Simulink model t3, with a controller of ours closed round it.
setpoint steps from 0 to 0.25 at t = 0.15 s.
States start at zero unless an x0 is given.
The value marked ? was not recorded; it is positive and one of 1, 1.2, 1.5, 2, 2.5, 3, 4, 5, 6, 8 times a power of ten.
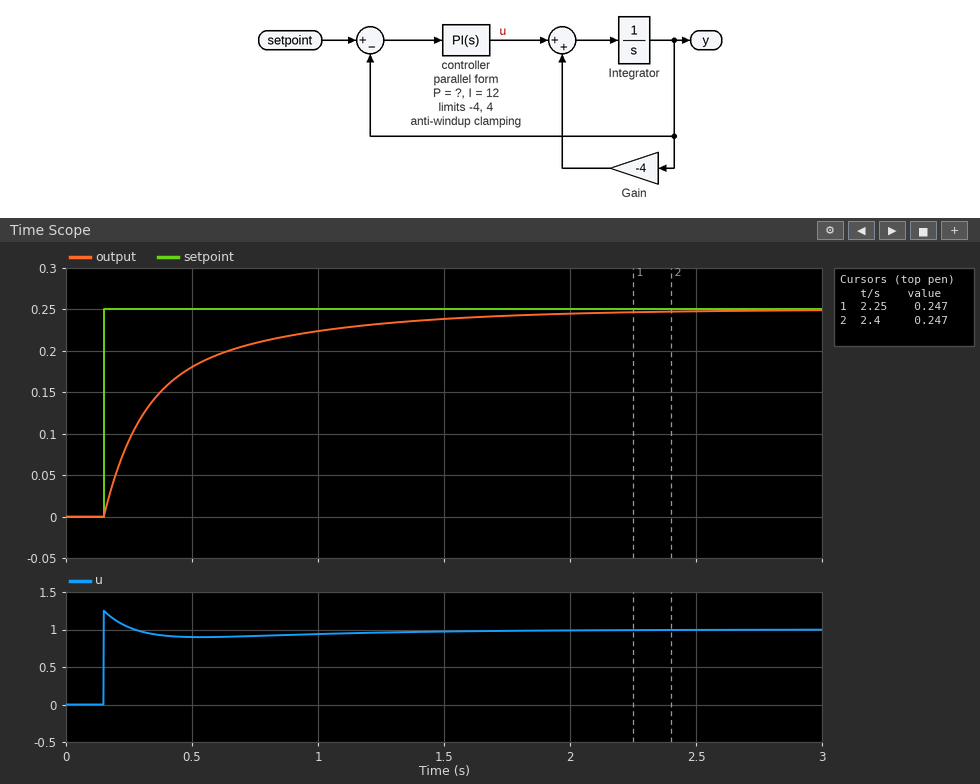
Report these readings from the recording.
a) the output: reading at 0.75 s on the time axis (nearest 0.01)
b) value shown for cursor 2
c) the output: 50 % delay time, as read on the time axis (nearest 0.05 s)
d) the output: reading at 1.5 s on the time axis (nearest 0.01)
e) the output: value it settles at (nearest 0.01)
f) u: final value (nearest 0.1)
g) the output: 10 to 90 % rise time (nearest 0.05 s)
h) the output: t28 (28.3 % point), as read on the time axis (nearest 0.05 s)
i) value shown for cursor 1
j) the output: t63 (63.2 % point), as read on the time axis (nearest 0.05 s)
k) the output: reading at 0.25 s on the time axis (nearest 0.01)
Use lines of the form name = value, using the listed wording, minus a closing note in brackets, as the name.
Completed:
the output: reading at 0.75 s on the time axis = 0.21
value shown for cursor 2 = 0.247
the output: 50 % delay time, as read on the time axis = 0.30 s
the output: reading at 1.5 s on the time axis = 0.24
the output: value it settles at = 0.25
u: final value = 1.0
the output: 10 to 90 % rise time = 0.85 s
the output: t28 (28.3 % point), as read on the time axis = 0.20 s
value shown for cursor 1 = 0.247
the output: t63 (63.2 % point), as read on the time axis = 0.40 s
the output: reading at 0.25 s on the time axis = 0.09
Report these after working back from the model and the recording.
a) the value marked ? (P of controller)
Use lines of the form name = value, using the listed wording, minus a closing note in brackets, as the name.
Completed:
the value marked ? = 5
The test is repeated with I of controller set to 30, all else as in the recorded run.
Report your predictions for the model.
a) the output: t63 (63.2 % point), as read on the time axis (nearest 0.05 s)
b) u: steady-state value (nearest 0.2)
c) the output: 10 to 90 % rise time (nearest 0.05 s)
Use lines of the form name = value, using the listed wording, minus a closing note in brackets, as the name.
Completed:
the output: t63 (63.2 % point), as read on the time axis = 0.30 s
u: steady-state value = 1.0
the output: 10 to 90 % rise time = 0.30 s
